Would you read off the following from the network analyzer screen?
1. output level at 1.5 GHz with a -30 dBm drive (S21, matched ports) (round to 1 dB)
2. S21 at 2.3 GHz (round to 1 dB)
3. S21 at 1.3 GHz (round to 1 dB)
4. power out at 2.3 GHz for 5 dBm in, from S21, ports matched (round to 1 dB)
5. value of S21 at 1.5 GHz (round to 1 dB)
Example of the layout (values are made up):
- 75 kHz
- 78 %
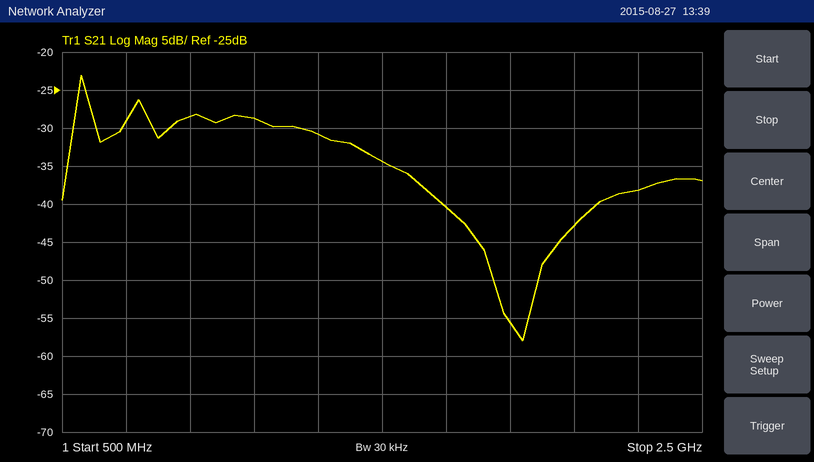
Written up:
- -64 dBm
- -38 dB
- -31 dB
- -33 dBm
- -34 dB
